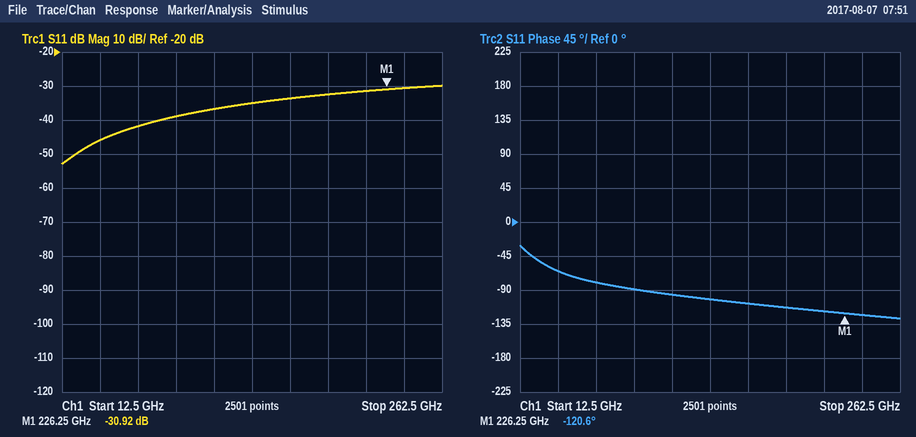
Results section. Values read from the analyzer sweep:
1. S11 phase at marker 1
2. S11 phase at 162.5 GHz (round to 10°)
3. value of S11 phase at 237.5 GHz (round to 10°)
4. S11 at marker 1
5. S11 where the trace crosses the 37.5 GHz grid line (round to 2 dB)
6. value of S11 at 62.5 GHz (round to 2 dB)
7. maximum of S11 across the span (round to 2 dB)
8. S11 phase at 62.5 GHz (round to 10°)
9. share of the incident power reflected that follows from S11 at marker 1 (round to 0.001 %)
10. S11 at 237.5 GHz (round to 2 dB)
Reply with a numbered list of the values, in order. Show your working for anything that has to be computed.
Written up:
1. -120.6°
2. -110°
3. -120°
4. -30.92 dB
5. -46 dB
6. -42 dB
7. -30 dB
8. -80°
9. 10^(-30.92/10) ≈ 0.081 %
10. -30 dB
